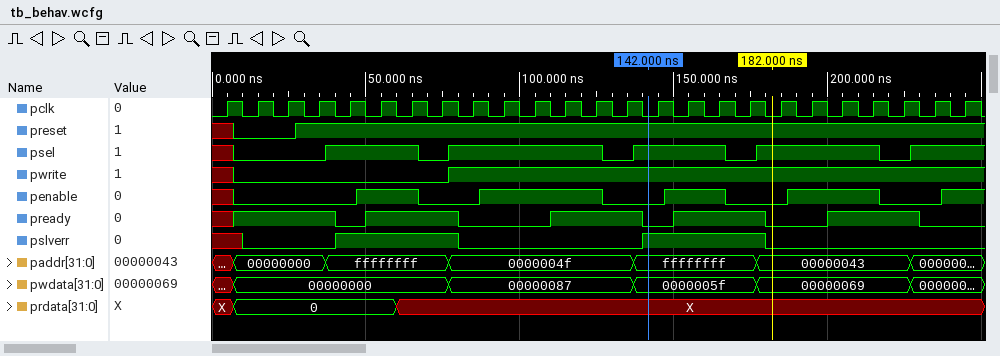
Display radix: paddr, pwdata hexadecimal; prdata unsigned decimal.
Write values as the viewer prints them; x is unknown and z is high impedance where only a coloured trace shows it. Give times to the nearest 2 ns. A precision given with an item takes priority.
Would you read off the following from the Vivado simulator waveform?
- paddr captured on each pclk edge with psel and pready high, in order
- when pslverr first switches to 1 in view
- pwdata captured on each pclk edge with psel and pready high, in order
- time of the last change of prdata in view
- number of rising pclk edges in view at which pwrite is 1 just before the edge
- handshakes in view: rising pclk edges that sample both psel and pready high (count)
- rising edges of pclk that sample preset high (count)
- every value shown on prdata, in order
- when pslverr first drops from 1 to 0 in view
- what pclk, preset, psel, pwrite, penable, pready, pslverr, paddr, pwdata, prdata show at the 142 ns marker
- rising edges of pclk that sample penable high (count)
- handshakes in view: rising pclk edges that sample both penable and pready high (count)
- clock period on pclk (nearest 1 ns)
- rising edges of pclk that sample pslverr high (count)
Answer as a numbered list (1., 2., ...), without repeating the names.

1. ffffffff, ffffffff, 0000004f, 0000004f, ffffffff, ffffffff, 00000043, 00000043
2. 40 ns
3. 00000000, 00000000, 00000087, 00000087, 0000005f, 0000005f, 00000069, 00000069
4. 60 ns
5. 17
6. 8
7. 22
8. X, 0, X
9. 80 ns
10. pclk=0, preset=1, psel=1, pwrite=1, penable=0, pready=0, pslverr=1, paddr=ffffffff, pwdata=0000005f, prdata=X
11. 12
12. 8
13. 10 ns
14. 8
